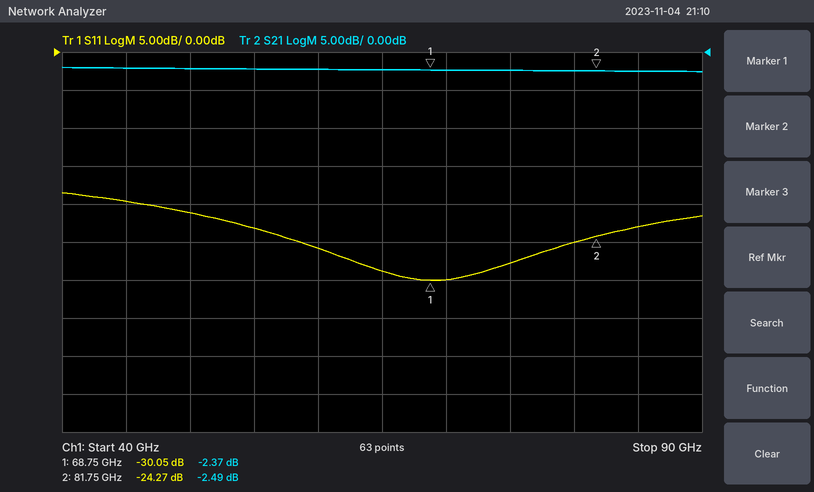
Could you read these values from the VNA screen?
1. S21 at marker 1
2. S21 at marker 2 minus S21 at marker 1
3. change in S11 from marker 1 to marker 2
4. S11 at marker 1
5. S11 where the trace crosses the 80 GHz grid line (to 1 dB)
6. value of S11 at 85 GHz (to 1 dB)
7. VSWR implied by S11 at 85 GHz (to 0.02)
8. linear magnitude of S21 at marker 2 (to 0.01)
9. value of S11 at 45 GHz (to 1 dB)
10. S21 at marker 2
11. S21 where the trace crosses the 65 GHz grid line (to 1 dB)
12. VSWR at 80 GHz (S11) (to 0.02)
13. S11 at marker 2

-2.37 dB
-0.12 dB
5.78 dB
-30.05 dB
-25 dB
-23 dB
1.16
0.75
-20 dB
-2.49 dB
-2 dB
1.12
-24.27 dB
